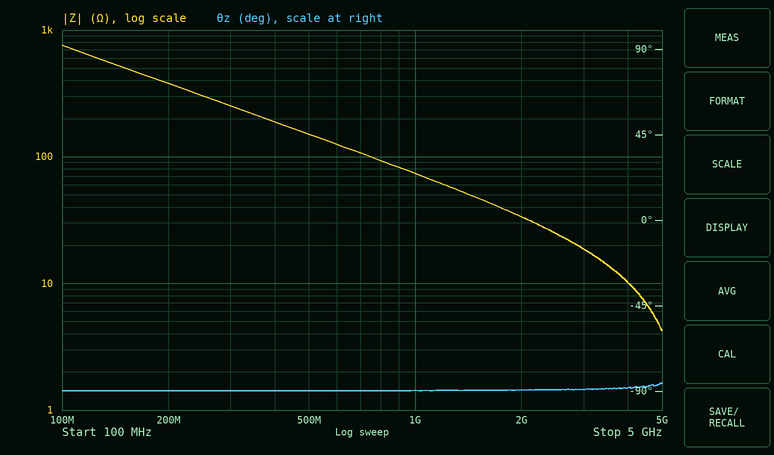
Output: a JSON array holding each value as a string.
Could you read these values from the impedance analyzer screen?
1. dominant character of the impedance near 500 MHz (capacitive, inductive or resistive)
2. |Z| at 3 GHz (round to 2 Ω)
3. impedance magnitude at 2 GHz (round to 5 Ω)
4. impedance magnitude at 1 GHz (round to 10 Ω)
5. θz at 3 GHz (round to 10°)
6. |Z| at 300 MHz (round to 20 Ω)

["capacitive", "18 Ω", "35 Ω", "70 Ω", "-90°", "260 Ω"]
